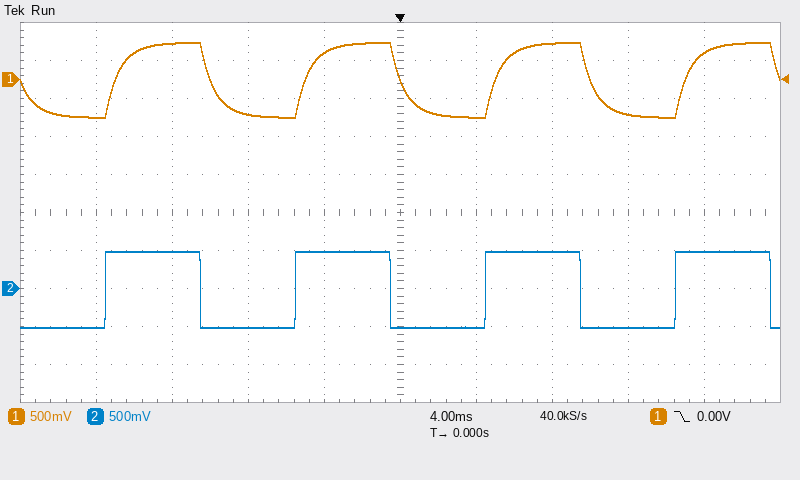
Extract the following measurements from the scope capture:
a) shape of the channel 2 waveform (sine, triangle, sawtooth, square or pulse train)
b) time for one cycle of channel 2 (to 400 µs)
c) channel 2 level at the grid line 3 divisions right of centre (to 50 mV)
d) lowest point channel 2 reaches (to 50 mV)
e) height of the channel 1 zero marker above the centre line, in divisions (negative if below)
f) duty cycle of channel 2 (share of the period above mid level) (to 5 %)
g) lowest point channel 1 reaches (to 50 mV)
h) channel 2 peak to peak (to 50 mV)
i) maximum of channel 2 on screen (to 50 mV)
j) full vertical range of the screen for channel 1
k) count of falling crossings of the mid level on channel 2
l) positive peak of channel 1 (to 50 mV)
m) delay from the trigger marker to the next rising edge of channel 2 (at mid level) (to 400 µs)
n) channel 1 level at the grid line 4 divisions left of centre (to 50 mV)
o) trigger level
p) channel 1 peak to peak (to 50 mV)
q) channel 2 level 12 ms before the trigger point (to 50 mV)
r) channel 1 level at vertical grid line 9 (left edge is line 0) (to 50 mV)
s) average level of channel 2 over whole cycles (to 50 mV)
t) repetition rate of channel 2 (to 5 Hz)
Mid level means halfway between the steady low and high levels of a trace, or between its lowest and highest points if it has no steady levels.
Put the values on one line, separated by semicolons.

square; 10.0 ms; -500 mV; -500 mV; +3.5 div; 50 %; -500 mV; 1.00 V; 500 mV; 5 V; 4; 500 mV; 4.4 ms; -500 mV; 0.00 V; 1.00 V; 500 mV; 350 mV; 0 mV; 100 Hz
